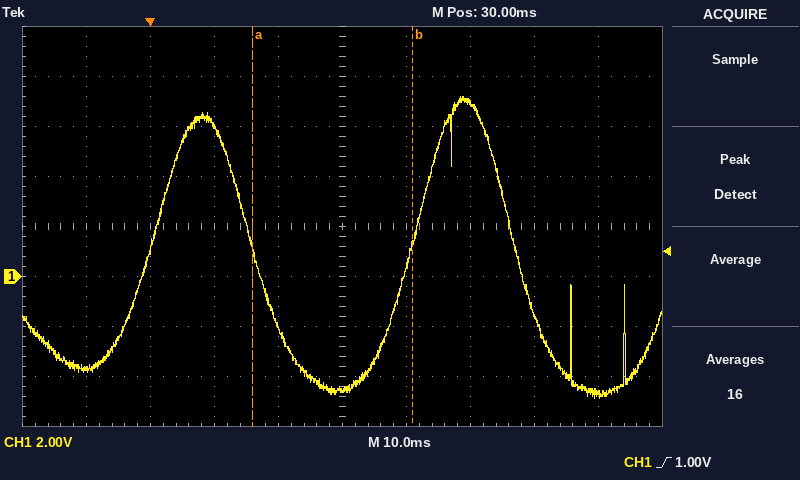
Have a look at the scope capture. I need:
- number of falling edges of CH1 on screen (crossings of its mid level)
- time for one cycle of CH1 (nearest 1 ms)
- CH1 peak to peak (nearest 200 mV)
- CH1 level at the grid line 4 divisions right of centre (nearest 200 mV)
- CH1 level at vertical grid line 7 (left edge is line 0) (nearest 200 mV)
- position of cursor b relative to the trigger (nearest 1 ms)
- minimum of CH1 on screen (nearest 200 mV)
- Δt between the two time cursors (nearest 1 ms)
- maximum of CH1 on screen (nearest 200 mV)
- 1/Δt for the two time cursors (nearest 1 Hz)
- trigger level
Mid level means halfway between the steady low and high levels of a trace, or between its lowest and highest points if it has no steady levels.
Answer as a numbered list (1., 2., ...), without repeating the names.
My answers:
1. 2
2. 41 ms
3. 12.0 V
4. -4.6 V
5. 7.0 V
6. +41 ms
7. -4.8 V
8. 25 ms
9. 7.2 V
10. 40 Hz
11. 1.00 V
